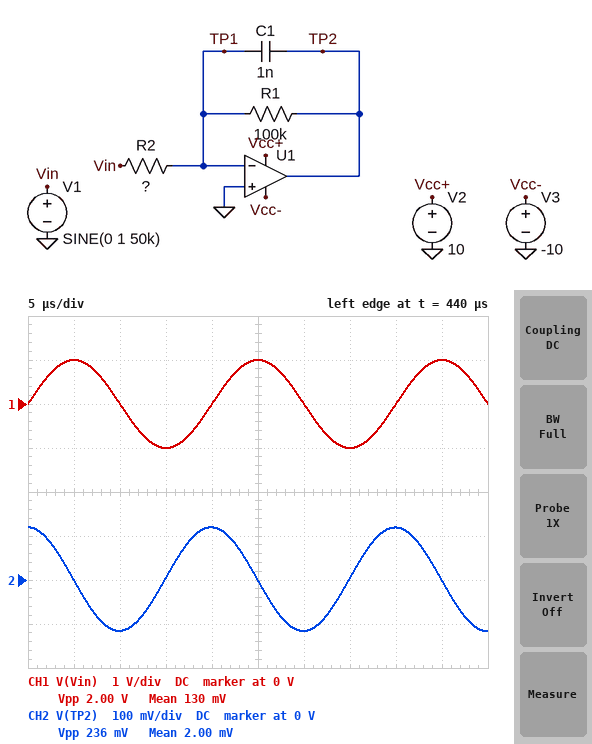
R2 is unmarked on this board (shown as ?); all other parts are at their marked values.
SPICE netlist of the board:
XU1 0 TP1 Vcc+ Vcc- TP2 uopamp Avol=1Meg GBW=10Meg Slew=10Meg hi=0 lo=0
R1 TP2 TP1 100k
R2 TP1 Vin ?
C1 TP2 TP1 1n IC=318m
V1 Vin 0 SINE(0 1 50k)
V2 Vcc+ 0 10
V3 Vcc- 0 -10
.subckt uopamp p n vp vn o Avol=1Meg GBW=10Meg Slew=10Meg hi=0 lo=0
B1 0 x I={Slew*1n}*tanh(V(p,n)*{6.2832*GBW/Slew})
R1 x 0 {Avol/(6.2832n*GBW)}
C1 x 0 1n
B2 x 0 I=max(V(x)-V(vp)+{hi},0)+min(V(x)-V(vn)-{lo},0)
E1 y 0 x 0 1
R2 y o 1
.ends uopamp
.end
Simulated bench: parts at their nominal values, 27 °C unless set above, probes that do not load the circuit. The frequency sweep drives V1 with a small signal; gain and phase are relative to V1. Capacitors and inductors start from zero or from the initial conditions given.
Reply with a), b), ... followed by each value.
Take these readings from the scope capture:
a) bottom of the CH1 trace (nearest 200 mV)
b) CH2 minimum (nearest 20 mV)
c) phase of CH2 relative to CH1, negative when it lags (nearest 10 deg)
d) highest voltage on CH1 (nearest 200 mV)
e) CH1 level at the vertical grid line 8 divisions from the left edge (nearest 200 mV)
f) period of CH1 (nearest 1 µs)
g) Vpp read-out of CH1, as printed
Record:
a) -1.0 V
b) -120 mV
c) 90 deg
d) 1.0 V
e) 0 V
f) 20 µs
g) 2.00 V
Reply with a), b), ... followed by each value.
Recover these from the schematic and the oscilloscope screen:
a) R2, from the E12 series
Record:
a) 27 kΩ
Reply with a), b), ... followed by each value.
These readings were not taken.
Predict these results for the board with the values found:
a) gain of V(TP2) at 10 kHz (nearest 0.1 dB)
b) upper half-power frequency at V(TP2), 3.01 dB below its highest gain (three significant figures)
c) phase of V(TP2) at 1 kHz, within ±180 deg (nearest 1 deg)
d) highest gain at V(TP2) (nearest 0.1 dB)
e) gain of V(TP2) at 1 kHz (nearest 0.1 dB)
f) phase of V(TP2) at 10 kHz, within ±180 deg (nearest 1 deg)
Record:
a) -4.7 dB
b) 1.59 kHz
c) 148 deg
d) 11.4 dB
e) 9.9 dB
f) 99 deg
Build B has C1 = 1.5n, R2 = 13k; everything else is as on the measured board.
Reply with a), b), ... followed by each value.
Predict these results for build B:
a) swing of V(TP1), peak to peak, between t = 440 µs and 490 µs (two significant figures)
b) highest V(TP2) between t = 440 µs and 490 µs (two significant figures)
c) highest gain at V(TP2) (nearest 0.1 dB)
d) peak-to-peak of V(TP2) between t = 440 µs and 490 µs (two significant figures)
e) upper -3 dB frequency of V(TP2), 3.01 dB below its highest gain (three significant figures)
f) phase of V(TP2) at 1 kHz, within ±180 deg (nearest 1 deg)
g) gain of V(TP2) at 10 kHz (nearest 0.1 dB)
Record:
a) 1.6 mV
b) 170 mV
c) 17.7 dB
d) 330 mV
e) 1.06 kHz
f) 137 deg
g) -1.8 dB
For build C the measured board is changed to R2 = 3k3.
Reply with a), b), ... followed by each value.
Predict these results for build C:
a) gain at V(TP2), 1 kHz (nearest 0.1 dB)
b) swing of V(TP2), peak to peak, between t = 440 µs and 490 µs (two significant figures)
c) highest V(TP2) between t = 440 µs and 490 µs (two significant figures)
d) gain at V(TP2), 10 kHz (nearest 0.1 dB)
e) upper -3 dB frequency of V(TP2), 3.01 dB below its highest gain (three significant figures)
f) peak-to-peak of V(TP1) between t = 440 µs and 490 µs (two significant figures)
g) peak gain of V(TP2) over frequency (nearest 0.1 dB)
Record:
a) 28.2 dB
b) 1.9 V
c) 950 mV
d) 13.5 dB
e) 1.58 kHz
f) 9.6 mV
g) 29.6 dB
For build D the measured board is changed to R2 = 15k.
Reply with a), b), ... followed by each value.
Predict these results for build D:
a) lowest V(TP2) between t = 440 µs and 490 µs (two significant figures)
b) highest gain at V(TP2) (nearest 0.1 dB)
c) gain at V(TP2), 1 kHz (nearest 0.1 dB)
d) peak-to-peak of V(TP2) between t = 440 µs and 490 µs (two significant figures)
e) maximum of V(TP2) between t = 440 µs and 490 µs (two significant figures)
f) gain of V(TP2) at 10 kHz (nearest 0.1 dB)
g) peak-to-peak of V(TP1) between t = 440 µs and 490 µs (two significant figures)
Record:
a) -210 mV
b) 16.5 dB
c) 15.0 dB
d) 420 mV
e) 210 mV
f) 0.4 dB
g) 2.1 mV
